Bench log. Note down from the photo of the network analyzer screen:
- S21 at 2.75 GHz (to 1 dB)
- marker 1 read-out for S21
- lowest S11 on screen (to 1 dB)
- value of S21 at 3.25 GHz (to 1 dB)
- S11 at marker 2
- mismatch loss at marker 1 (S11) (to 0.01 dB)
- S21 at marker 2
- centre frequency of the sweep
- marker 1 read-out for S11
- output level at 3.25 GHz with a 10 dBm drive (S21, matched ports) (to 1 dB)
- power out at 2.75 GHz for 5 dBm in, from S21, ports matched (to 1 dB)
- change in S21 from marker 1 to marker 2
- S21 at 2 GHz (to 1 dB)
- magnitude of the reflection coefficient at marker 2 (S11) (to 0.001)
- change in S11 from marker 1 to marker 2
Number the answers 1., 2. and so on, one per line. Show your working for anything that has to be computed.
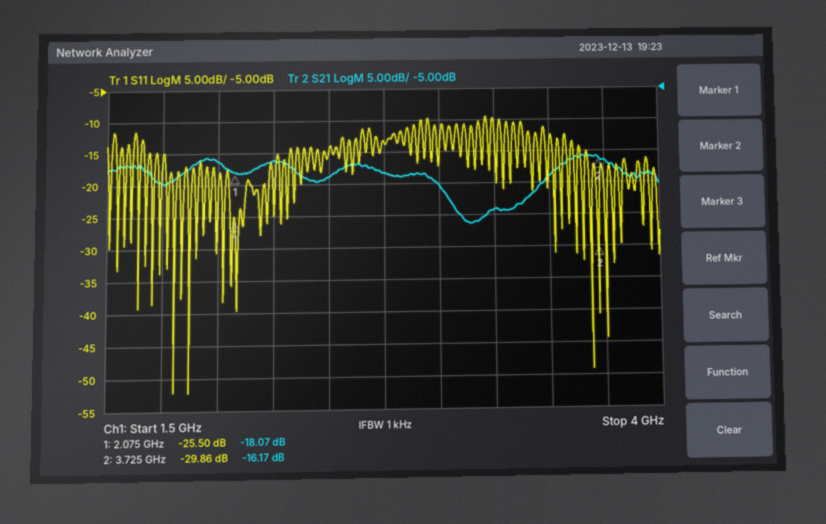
1. -18 dB
2. -18.07 dB
3. -52 dB
4. -24 dB
5. -29.86 dB
6. −10 log10(1 − 10^(-25.5/10)) ≈ 0.01 dB
7. -16.17 dB
8. 2.75 GHz
9. -25.50 dB
10. 10 dBm + (-24 dB) = -14 dBm
11. 5 dBm + (-18 dB) = -13 dBm
12. -16.17 − (-18.07) = 1.90 dB
13. -16 dB
14. 10^(-29.86/20) ≈ 0.032
15. -29.86 − (-25.5) = -4.36 dB
